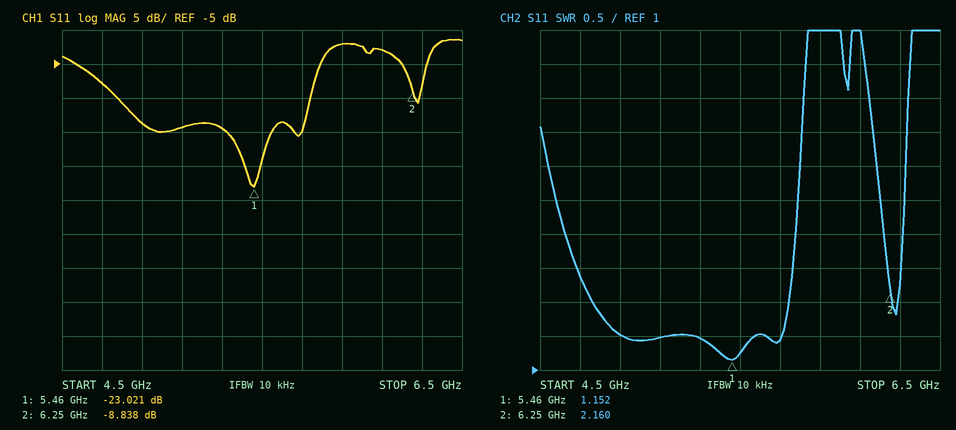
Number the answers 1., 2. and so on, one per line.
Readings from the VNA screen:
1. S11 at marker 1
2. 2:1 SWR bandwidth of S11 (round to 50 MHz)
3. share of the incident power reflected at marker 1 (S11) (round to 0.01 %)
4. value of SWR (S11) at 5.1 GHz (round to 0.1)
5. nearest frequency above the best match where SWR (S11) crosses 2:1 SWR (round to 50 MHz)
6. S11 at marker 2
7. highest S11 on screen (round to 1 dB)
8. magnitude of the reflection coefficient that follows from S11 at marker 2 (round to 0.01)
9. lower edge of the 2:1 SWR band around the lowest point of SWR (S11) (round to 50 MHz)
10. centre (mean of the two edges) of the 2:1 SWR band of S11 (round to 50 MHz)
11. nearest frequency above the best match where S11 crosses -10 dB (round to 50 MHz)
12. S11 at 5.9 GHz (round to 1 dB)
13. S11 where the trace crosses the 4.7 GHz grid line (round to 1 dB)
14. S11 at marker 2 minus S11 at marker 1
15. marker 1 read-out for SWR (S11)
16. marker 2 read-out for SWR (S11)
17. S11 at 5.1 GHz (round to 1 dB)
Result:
1. -23.021 dB
2. 1.00 GHz
3. 0.50 %
4. 1.5
5. 5.75 GHz
6. -8.838 dB
7. -1 dB
8. 0.36
9. 4.75 GHz
10. 5.25 GHz
11. 5.75 GHz
12. -2 dB
13. -8 dB
14. 14.183 dB
15. 1.152
16. 2.160
17. -14 dB
